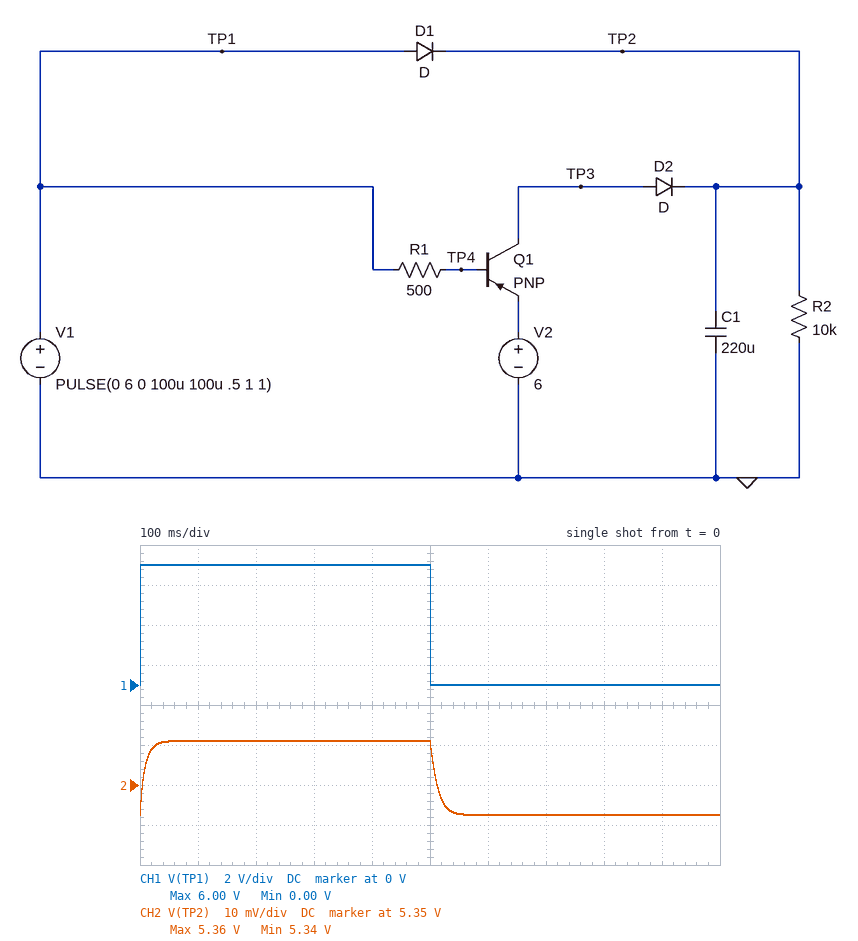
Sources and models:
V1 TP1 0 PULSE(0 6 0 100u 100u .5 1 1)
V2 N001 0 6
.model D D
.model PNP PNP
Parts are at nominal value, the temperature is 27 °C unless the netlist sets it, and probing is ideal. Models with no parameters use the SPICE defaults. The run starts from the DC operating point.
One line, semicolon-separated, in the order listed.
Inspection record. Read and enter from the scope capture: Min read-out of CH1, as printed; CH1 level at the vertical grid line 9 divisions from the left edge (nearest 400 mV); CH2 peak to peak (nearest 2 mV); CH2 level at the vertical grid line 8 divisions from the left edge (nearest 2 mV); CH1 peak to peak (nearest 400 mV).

0.00 V; 0 V; 18 mV; 5.342 V; 6.0 V
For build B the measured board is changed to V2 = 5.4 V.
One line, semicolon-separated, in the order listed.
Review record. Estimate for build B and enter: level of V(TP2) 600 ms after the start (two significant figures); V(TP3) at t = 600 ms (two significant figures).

5.1 V; 5.4 V
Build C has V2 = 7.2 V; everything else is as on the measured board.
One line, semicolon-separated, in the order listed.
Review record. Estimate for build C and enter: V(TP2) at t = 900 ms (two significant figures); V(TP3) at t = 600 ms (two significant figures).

6.5 V; 7.2 V
